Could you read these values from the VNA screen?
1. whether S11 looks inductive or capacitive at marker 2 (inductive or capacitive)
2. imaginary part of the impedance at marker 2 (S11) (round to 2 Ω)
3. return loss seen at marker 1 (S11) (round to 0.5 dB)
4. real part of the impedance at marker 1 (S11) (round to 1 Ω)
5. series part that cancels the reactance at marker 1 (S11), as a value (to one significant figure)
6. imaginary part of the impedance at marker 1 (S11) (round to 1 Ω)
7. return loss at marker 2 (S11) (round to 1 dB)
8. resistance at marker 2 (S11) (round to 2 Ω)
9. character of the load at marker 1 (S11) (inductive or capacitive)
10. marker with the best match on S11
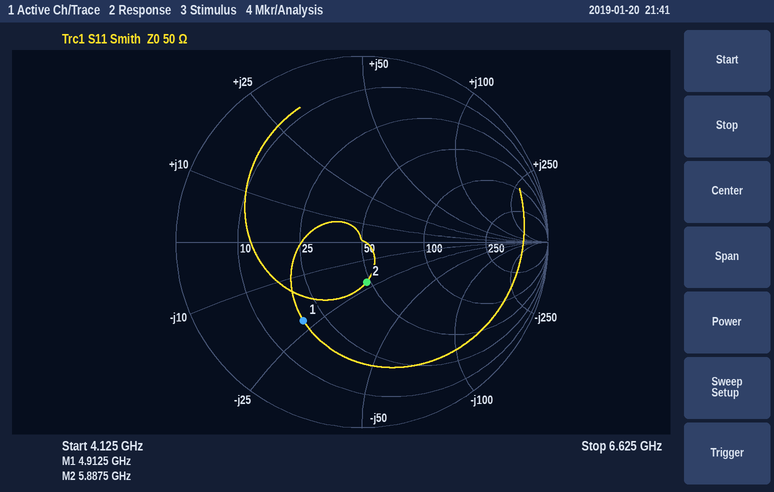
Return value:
capacitive
-22 Ω
5.5 dB
19 Ω
700 pH
-22 Ω
13 dB
48 Ω
capacitive
marker 2
